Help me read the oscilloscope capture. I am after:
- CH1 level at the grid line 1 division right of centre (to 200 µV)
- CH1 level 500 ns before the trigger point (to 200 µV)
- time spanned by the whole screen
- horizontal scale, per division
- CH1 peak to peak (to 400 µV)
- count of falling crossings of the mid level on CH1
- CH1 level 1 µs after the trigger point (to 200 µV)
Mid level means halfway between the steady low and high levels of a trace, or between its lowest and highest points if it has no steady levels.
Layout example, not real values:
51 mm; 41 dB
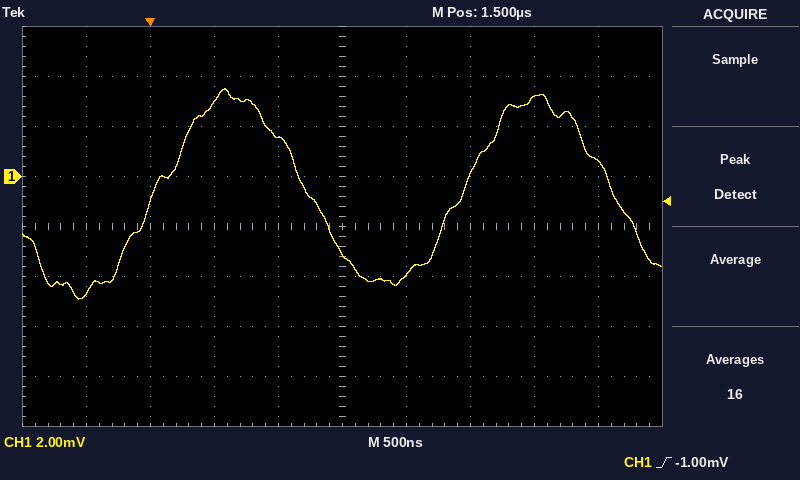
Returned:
-4.0 mV; -4.6 mV; 5 µs; 500 ns; 8.4 mV; 2; 1.6 mV
